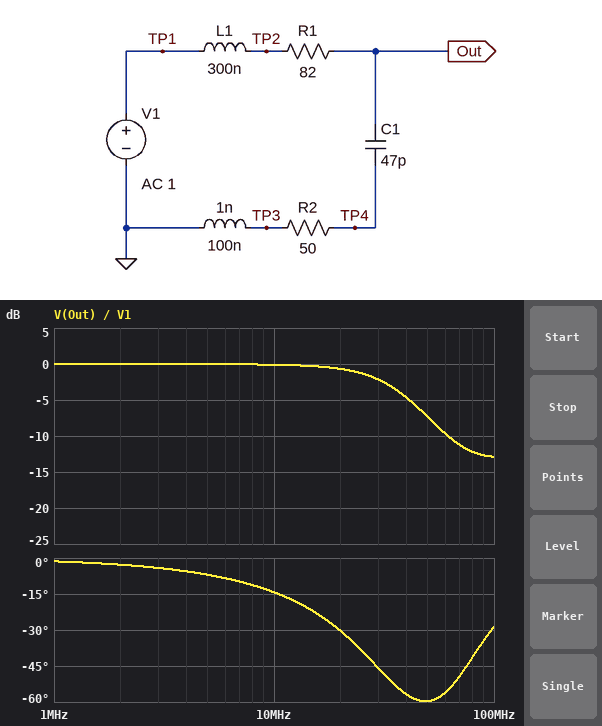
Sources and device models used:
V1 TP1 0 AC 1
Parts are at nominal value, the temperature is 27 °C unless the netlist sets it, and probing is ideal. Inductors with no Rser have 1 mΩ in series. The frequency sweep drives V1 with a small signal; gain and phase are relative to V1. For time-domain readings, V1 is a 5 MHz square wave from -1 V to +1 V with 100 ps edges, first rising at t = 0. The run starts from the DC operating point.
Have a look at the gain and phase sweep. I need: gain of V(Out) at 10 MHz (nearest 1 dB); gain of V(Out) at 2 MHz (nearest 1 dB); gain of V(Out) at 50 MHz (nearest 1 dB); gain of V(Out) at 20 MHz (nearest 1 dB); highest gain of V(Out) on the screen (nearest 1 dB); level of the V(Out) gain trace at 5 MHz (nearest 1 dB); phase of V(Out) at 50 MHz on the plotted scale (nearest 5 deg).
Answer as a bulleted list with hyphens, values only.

- 0 dB
- 0 dB
- -7 dB
- -1 dB
- 0 dB
- 0 dB
- -60 deg
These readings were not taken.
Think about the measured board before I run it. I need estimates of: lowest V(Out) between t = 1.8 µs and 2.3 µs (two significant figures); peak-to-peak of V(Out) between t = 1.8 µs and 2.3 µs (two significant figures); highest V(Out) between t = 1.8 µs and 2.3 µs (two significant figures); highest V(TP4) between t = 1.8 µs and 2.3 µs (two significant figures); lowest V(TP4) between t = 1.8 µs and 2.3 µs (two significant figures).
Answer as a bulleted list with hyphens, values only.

- -1.1 V
- 2.1 V
- 1.1 V
- 580 mV
- -580 mV
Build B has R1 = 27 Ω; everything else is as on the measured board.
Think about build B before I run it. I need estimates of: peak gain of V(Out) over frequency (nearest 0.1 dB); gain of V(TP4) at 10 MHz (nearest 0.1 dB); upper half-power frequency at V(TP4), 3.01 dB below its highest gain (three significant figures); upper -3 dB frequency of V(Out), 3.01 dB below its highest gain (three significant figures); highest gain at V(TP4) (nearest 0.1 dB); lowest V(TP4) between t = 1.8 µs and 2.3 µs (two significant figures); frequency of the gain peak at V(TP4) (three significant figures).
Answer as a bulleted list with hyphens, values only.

- 1.9 dB
- -16.1 dB
- 60.9 MHz
- 42.8 MHz
- -2.9 dB
- -730 mV
- 37.9 MHz
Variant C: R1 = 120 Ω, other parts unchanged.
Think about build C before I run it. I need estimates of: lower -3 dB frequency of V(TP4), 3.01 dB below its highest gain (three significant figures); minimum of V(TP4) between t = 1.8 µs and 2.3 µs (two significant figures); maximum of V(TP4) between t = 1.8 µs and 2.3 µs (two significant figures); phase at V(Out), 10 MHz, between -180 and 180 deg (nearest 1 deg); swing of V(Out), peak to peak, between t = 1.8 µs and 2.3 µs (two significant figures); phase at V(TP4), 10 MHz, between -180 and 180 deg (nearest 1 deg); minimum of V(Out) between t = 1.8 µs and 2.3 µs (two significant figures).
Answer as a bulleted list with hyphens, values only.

- 18.3 MHz
- -520 mV
- 520 mV
- -20 deg
- 2.0 V
- 69 deg
- -1.0 V
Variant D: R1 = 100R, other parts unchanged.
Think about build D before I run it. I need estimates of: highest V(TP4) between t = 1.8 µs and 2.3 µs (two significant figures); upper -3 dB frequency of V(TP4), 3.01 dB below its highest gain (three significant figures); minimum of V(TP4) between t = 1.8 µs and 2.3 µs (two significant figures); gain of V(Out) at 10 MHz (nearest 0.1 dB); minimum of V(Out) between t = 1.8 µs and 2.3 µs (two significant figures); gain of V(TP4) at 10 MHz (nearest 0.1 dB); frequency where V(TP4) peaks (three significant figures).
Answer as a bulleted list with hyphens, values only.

- 550 mV
- 224 MHz
- -550 mV
- -0.3 dB
- -1.0 V
- -16.8 dB
- 42.7 MHz
